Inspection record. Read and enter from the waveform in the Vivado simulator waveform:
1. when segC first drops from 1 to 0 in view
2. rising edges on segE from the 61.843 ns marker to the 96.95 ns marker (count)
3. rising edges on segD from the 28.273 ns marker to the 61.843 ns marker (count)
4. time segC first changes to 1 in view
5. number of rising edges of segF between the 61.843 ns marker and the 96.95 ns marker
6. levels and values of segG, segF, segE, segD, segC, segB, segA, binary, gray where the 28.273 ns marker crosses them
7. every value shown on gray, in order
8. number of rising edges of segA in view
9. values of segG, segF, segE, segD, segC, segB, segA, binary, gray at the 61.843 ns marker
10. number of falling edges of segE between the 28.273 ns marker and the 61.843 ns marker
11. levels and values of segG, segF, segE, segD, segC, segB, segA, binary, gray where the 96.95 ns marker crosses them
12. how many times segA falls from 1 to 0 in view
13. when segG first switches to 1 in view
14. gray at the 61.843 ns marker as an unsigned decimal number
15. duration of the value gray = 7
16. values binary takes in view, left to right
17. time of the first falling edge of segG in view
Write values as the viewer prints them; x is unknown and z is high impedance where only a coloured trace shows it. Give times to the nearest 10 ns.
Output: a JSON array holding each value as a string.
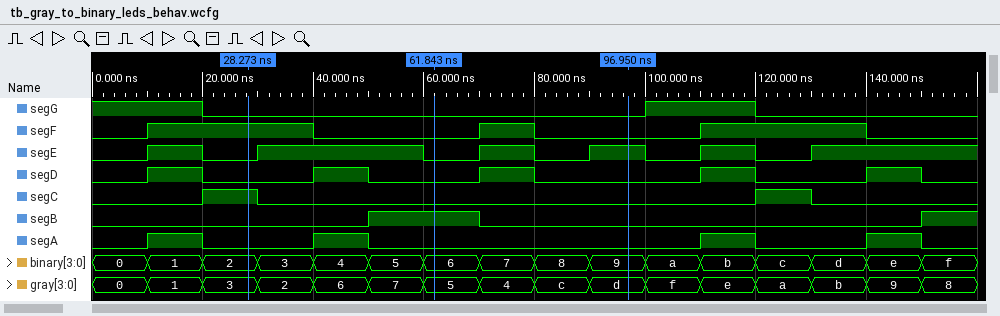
["30 ns", "2", "1", "20 ns", "1", "segG=0, segF=1, segE=0, segD=0, segC=1, segB=0, segA=0, binary=2, gray=3", "0, 1, 3, 2, 6, 7, 5, 4, c, d, f, e, a, b, 9, 8", "4", "segG=0, segF=0, segE=0, segD=0, segC=0, segB=1, segA=0, binary=6, gray=5", "1", "segG=0, segF=0, segE=1, segD=0, segC=0, segB=0, segA=0, binary=9, gray=d", "4", "100 ns", "5", "10 ns", "0, 1, 2, 3, 4, 5, 6, 7, 8, 9, a, b, c, d, e, f", "20 ns"]
